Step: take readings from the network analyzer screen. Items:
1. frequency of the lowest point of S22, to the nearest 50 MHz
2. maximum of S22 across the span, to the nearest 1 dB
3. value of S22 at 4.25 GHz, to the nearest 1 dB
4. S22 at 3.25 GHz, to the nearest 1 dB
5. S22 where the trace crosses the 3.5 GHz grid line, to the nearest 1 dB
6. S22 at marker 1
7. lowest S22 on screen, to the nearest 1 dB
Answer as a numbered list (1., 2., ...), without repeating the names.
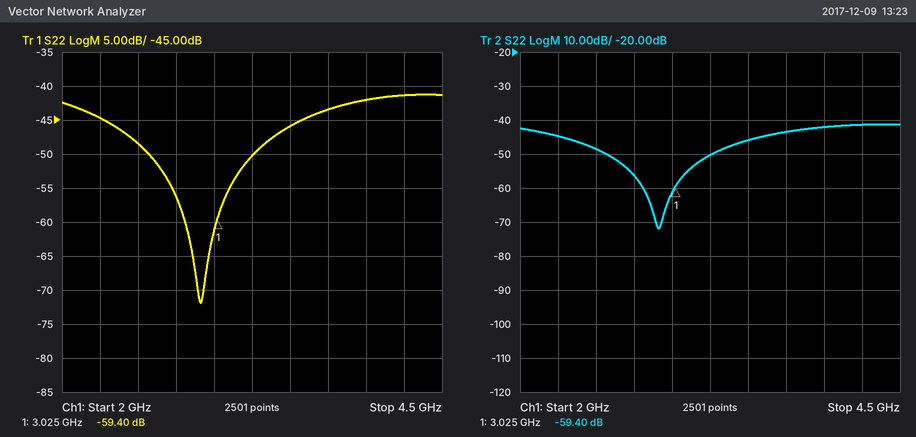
1. 2.90 GHz
2. -41 dB
3. -41 dB
4. -50 dB
5. -46 dB
6. -59.40 dB
7. -72 dB
